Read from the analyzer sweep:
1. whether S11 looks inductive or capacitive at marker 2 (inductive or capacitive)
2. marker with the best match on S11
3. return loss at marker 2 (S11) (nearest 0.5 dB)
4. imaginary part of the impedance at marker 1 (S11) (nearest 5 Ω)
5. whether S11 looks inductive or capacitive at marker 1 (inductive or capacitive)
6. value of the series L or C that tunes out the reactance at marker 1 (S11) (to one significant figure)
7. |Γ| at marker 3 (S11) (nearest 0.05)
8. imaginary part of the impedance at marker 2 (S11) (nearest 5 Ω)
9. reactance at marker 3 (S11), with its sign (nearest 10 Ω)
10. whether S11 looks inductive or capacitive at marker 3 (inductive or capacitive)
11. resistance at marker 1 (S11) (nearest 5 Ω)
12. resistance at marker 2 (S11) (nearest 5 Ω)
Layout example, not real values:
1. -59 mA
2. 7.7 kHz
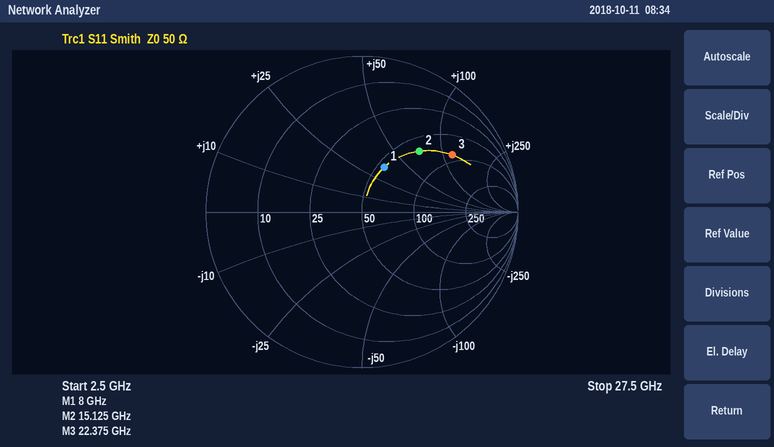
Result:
1. inductive
2. marker 1
3. 5.5 dB
4. +35 Ω
5. inductive
6. 600 fF
7. 0.70
8. +70 Ω
9. +120 Ω
10. inductive
11. 55 Ω
12. 65 Ω
